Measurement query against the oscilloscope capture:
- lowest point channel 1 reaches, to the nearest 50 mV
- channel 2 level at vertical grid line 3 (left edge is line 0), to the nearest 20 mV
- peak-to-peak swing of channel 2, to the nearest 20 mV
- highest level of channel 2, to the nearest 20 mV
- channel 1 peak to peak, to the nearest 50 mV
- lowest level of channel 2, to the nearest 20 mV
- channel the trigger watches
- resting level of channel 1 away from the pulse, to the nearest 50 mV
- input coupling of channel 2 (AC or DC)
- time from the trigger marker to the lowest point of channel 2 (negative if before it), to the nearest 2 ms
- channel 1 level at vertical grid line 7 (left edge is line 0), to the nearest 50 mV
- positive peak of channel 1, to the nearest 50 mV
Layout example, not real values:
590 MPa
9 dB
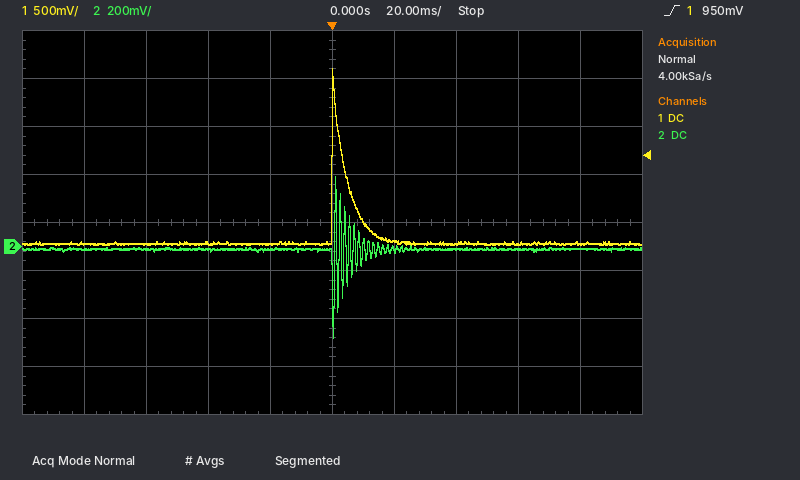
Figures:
0 mV
-20 mV
680 mV
300 mV
1.85 V
-380 mV
channel 1
50 mV
DC
0 ms
50 mV
1.85 V
